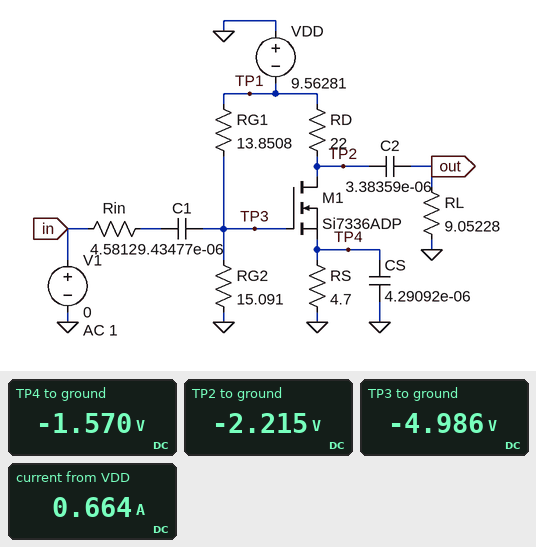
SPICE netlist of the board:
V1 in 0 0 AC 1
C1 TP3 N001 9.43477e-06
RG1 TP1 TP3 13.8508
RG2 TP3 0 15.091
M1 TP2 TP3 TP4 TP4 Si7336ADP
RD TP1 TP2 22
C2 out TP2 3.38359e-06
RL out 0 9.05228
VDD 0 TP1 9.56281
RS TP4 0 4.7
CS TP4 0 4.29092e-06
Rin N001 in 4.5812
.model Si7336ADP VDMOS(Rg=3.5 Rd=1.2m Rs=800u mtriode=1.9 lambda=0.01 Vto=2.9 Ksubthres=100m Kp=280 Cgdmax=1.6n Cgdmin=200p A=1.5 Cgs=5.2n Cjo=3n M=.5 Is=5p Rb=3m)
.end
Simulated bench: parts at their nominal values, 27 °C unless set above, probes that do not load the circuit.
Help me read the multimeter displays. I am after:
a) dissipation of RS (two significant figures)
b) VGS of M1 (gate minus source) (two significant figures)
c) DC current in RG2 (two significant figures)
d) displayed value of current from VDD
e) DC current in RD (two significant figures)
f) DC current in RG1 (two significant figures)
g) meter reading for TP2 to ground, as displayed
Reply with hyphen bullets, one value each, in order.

- 520 mW
- -3.4 V
- 330 mA
- 0.664 A
- 330 mA
- 330 mA
- -2.215 V
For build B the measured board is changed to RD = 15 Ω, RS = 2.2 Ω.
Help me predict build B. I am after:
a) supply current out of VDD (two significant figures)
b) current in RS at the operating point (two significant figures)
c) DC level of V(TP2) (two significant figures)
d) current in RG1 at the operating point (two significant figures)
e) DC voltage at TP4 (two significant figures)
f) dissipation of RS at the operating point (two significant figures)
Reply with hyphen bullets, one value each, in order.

- 850 mA
- 520 mA
- -1.8 V
- 330 mA
- -1.1 V
- 590 mW
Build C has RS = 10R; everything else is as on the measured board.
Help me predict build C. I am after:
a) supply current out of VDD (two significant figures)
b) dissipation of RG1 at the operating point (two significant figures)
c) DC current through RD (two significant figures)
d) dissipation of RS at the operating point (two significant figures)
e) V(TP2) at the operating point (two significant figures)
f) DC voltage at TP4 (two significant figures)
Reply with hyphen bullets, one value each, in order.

- 610 mA
- 1.5 W
- 280 mA
- 780 mW
- -3.4 V
- -2.8 V
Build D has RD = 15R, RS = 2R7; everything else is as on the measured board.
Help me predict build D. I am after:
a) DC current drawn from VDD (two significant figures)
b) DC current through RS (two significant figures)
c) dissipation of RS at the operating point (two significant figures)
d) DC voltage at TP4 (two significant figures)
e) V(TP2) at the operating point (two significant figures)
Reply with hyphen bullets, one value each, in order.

- 830 mA
- 500 mA
- 680 mW
- -1.4 V
- -2.0 V
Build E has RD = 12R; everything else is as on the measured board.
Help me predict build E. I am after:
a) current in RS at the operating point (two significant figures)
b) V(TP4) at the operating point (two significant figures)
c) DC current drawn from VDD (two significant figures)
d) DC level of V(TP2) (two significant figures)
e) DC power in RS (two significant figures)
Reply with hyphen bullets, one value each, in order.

- 530 mA
- -2.5 V
- 860 mA
- -3.2 V
- 1.3 W
